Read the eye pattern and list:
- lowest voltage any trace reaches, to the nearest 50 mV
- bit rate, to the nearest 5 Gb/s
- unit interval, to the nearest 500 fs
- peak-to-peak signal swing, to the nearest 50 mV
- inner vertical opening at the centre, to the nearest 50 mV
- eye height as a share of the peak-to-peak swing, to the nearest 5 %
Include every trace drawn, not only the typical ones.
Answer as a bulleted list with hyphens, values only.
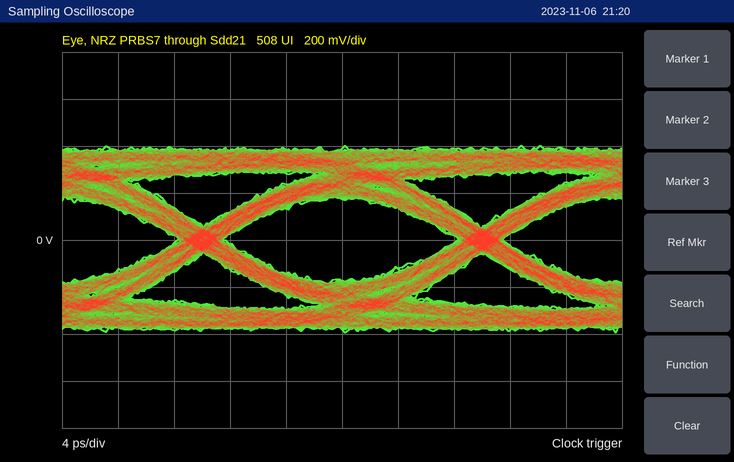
- -400 mV
- 50 Gb/s
- 20.0 ps
- 800 mV
- 350 mV
- 45 %
